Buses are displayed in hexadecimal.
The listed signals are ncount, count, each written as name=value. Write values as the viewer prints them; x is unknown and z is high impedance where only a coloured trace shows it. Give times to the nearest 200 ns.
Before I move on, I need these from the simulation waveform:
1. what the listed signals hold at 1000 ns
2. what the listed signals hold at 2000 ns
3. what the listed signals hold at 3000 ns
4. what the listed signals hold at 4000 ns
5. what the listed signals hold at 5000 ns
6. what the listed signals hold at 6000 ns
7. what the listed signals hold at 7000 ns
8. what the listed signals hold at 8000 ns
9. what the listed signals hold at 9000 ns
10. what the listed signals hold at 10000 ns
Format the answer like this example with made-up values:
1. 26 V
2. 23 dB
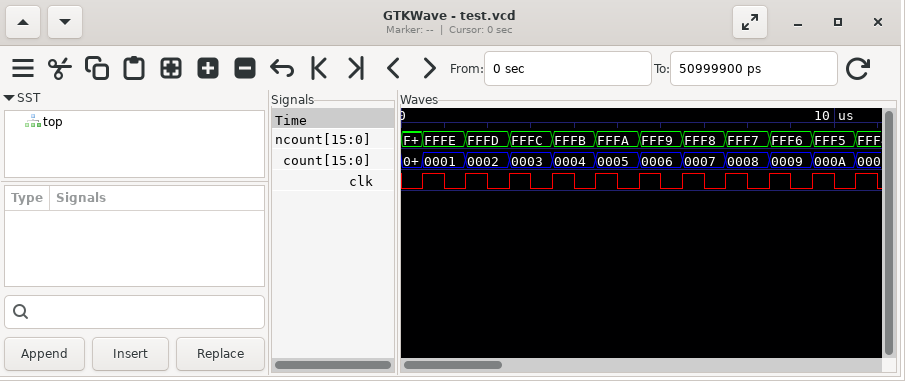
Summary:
1. ncount=FFFE, count=0001
2. ncount=FFFD, count=0002
3. ncount=FFFC, count=0003
4. ncount=FFFB, count=0004
5. ncount=FFFA, count=0005
6. ncount=FFF9, count=0006
7. ncount=FFF8, count=0007
8. ncount=FFF7, count=0008
9. ncount=FFF6, count=0009
10. ncount=FFF5, count=000A
